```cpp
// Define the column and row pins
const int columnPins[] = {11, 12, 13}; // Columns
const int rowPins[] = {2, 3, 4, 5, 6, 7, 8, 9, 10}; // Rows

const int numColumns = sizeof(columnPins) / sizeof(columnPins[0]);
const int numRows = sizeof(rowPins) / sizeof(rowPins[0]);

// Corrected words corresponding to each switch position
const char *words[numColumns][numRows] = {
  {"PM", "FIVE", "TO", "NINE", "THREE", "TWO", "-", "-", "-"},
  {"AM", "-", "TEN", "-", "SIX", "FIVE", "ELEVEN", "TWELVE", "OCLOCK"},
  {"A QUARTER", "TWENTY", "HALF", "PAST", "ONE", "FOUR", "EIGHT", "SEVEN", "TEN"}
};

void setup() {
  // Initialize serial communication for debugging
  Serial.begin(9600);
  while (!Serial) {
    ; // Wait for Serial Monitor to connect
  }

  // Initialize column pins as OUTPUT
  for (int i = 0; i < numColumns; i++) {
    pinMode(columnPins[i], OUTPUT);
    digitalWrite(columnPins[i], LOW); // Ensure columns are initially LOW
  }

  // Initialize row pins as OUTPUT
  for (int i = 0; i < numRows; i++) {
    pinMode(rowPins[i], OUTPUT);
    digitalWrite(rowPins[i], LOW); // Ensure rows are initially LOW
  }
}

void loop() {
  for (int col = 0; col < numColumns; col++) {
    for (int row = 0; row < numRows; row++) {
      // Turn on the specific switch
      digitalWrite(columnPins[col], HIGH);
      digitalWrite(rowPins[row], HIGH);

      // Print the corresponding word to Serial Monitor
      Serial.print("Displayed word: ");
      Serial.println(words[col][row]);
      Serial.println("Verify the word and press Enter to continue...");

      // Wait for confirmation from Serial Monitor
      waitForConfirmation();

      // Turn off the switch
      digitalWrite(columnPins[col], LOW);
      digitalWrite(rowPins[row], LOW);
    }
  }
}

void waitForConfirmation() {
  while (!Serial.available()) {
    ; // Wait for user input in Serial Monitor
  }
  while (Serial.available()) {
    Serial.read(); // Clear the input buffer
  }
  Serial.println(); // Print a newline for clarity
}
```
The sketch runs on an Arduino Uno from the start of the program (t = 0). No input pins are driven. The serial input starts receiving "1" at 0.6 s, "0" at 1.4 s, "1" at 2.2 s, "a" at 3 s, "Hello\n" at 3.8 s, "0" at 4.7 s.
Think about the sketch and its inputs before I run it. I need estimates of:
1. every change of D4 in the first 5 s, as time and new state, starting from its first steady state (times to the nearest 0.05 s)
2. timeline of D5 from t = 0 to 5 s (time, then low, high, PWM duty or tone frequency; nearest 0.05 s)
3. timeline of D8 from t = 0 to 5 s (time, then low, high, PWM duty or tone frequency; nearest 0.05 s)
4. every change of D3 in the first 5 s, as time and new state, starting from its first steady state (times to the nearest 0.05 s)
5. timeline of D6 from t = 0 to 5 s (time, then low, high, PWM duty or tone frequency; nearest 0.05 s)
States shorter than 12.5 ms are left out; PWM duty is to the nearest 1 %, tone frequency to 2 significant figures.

0 s low; 1.4 s high; 2.2 s low
0 s low; 2.2 s high; 3 s low
0 s low; 3.8 s high; 4.7 s low
0 s low; 0.6 s high; 1.4 s low
0 s low; 3 s high; 3.8 s low
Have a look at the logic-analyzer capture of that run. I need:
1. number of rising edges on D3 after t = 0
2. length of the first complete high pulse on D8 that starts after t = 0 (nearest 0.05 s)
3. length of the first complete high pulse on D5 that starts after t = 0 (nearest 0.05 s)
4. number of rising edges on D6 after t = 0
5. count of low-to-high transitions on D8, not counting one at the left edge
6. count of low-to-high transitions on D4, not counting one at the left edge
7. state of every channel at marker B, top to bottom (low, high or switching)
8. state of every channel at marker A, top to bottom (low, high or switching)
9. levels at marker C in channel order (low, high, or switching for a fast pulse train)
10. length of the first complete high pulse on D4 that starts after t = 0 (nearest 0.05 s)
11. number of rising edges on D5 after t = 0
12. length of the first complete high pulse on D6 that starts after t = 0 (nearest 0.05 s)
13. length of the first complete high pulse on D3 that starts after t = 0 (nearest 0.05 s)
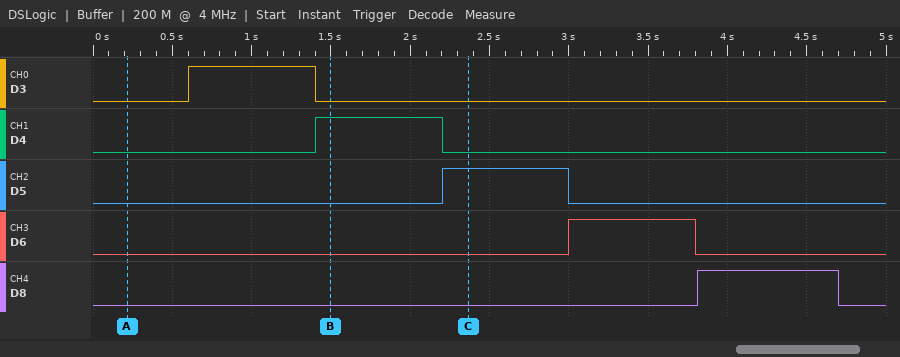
1
0.90 s
0.80 s
1
1
1
D3 low, D4 high, D5 low, D6 low, D8 low
D3 low, D4 low, D5 low, D6 low, D8 low
D3 low, D4 low, D5 high, D6 low, D8 low
0.80 s
1
0.80 s
0.80 s
